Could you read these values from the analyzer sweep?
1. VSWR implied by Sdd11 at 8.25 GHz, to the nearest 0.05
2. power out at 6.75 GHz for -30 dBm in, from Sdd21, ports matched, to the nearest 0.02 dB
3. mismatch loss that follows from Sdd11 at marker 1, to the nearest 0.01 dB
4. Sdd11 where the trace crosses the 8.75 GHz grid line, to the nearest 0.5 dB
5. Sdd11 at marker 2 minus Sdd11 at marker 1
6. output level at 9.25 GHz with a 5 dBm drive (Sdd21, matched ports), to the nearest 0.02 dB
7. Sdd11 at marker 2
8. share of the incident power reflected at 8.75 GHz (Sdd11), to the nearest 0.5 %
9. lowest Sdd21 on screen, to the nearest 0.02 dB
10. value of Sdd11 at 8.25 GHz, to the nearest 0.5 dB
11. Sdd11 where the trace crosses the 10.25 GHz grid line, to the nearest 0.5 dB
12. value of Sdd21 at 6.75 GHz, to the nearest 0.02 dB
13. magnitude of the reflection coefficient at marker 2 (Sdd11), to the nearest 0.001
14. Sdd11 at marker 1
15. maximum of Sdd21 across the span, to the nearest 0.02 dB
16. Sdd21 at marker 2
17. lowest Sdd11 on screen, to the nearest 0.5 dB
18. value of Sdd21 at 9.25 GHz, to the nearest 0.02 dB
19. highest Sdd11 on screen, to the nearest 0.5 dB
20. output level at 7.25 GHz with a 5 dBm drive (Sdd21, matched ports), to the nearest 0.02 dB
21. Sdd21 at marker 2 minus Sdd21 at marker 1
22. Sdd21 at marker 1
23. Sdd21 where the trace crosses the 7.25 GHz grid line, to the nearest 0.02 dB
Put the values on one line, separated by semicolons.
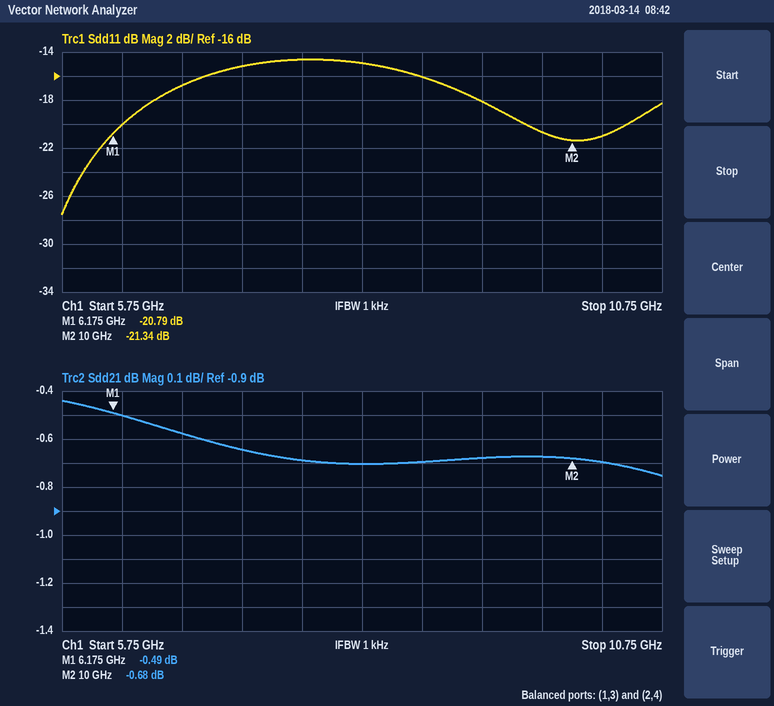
1.45; -30.58 dBm; 0.04 dB; -16.0 dB; -0.55 dB; 4.32 dBm; -21.34 dB; 2.5 %; -0.76 dB; -15.0 dB; -21.0 dB; -0.58 dB; 0.086; -20.79 dB; -0.44 dB; -0.68 dB; -27.5 dB; -0.68 dB; -14.5 dB; 4.36 dBm; -0.19 dB; -0.49 dB; -0.64 dB
